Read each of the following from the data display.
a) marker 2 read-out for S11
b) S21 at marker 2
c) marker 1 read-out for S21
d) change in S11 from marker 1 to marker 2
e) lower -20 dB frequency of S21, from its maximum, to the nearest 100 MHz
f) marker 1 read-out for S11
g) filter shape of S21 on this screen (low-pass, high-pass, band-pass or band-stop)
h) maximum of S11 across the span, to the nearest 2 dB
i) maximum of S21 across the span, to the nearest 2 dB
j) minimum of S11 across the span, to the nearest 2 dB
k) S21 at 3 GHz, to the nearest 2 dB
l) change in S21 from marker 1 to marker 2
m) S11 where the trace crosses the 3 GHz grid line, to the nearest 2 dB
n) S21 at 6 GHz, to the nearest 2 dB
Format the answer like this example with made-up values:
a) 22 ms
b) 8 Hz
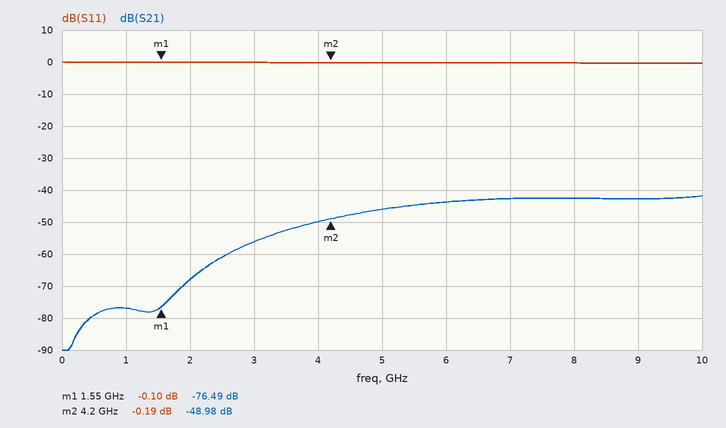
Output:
a) -0.19 dB
b) -48.98 dB
c) -76.49 dB
d) -0.09 dB
e) 2.4 GHz
f) -0.10 dB
g) high-pass
h) 0 dB
i) -42 dB
j) 0 dB
k) -56 dB
l) 27.51 dB
m) 0 dB
n) -44 dB
